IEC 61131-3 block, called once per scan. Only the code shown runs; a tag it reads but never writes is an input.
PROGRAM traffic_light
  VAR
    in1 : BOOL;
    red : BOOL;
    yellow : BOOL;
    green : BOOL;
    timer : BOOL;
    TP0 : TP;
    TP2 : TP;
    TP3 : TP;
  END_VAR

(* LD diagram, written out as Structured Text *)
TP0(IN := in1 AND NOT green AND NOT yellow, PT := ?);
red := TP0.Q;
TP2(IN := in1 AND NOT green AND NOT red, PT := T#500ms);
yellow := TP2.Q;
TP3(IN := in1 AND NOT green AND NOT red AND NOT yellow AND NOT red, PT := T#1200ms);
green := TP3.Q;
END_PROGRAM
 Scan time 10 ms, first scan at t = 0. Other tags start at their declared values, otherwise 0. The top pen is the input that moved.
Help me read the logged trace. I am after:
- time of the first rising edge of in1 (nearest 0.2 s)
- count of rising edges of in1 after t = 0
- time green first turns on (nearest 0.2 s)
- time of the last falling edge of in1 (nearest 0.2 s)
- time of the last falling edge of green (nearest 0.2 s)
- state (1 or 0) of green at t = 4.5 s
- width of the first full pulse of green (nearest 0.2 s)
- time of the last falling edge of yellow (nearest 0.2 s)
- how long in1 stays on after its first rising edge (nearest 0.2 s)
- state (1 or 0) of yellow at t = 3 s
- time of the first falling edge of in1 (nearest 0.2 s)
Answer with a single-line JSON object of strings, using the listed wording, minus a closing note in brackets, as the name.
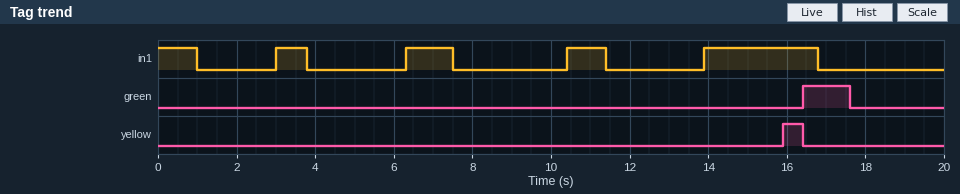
{"time of the first rising edge of in1": "3.0 s", "count of rising edges of in1 after t = 0": "4", "time green first turns on": "16.4 s", "time of the last falling edge of in1": "16.8 s", "time of the last falling edge of green": "17.6 s", "state (1 or 0) of green at t = 4.5 s": "0", "width of the first full pulse of green": "1.2 s", "time of the last falling edge of yellow": "16.4 s", "how long in1 stays on after its first rising edge": "0.8 s", "state (1 or 0) of yellow at t = 3 s": "0", "time of the first falling edge of in1": "1.0 s"}
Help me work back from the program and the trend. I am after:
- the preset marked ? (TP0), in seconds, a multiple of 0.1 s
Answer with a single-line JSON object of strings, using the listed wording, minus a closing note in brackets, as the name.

{"the preset marked ? (TP0), in seconds, a multiple of 0.1 s": "2.0 s"}
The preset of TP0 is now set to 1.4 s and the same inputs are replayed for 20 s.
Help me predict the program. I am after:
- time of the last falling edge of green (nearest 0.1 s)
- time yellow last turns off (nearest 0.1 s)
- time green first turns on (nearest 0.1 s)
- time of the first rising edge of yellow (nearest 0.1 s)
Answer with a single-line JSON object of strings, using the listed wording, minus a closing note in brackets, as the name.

{"time of the last falling edge of green": "17.0 s", "time yellow last turns off": "15.8 s", "time green first turns on": "15.8 s", "time of the first rising edge of yellow": "15.3 s"}
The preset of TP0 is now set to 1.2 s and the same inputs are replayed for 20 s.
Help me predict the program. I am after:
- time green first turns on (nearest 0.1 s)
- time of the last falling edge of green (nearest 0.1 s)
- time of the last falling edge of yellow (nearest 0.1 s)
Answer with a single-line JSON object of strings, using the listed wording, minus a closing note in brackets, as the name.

{"time green first turns on": "15.6 s", "time of the last falling edge of green": "16.8 s", "time of the last falling edge of yellow": "15.6 s"}
